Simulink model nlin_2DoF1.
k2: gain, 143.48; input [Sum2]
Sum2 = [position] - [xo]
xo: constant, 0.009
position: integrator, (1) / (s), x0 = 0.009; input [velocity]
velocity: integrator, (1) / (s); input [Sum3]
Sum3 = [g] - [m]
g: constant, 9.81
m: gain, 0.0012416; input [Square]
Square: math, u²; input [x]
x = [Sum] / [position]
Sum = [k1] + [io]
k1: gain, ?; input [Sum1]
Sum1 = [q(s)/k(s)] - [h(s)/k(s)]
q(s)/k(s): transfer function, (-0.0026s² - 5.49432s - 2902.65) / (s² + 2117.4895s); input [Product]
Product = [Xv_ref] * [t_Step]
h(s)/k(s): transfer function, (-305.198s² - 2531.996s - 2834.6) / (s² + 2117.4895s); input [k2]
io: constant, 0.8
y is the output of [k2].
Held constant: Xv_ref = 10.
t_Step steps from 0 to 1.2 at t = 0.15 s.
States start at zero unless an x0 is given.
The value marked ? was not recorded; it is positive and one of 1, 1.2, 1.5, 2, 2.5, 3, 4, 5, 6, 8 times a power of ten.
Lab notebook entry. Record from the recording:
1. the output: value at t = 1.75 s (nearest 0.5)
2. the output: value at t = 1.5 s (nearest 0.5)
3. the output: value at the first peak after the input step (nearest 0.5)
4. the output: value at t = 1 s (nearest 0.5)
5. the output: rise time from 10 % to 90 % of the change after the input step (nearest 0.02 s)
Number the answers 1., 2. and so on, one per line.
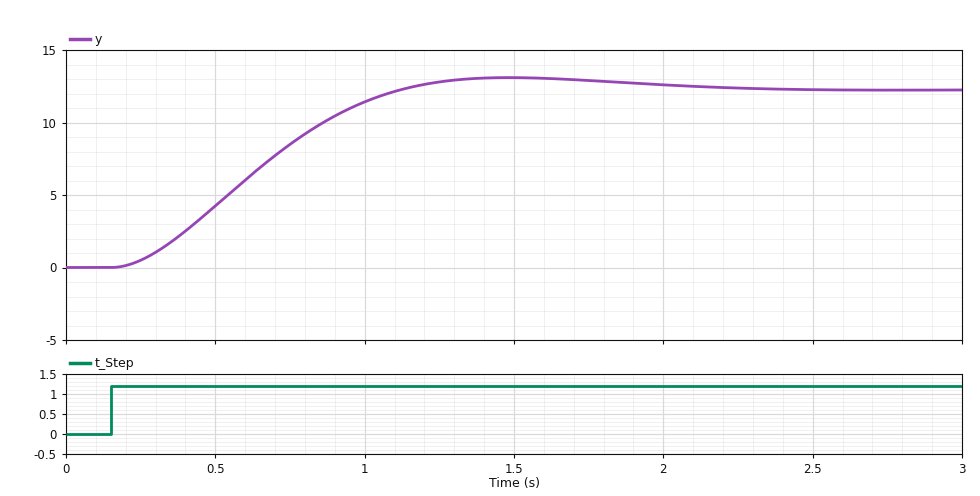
1. 13.0
2. 13.0
3. 13.0
4. 11.5
5. 0.64 s
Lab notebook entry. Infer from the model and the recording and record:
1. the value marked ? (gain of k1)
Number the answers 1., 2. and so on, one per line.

1. 1
